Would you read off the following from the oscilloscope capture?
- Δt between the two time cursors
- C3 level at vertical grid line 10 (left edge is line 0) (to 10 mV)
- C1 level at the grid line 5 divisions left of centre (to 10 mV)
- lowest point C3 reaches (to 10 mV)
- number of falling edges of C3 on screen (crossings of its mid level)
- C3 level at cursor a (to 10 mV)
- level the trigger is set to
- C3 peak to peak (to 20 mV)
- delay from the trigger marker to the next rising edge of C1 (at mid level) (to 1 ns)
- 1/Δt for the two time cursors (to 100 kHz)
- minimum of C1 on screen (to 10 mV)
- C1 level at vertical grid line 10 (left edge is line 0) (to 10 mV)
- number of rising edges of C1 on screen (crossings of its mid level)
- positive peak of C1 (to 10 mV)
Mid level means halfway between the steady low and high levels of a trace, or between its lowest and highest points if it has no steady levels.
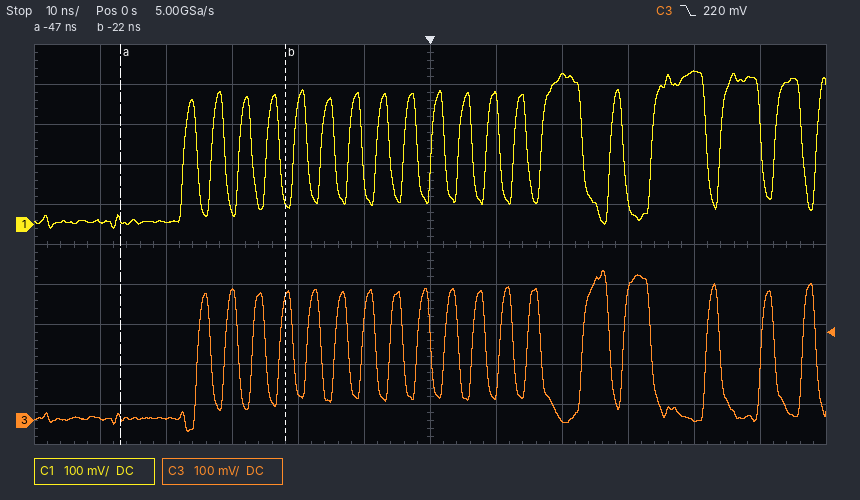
25 ns
0 mV
10 mV
-30 mV
18
10 mV
220 mV
400 mV
4 ns
40.0 MHz
-10 mV
380 mV
19
380 mV
